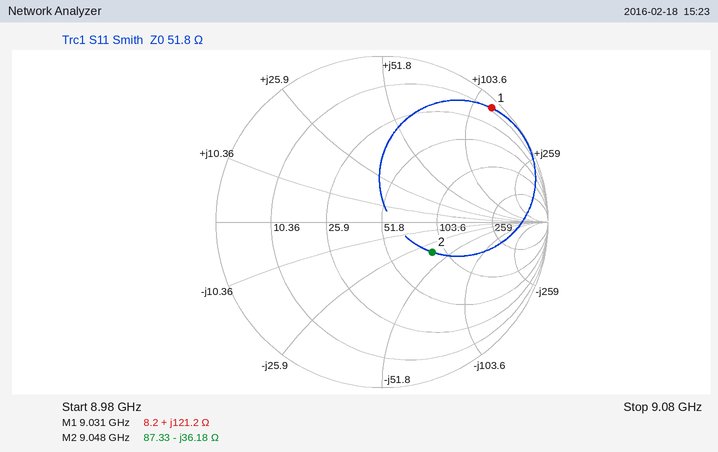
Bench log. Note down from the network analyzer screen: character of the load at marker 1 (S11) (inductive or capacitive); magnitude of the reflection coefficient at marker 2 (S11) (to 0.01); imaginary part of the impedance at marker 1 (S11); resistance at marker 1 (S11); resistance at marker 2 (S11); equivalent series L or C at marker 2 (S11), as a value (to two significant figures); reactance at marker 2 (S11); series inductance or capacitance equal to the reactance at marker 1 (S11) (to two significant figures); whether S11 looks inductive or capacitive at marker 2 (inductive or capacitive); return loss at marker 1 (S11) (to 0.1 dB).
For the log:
inductive
0.35
+121.2 Ω
8.2 Ω
87.33 Ω
490 fF
-36.18 Ω
2.1 nH
capacitive
0.4 dB
